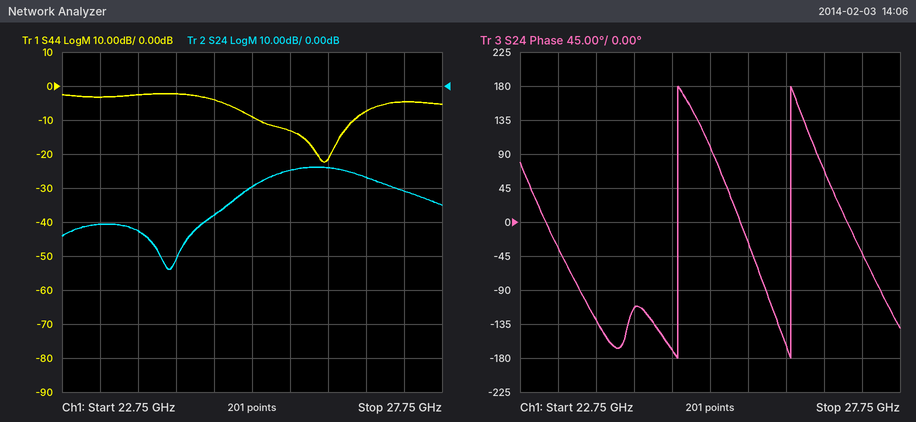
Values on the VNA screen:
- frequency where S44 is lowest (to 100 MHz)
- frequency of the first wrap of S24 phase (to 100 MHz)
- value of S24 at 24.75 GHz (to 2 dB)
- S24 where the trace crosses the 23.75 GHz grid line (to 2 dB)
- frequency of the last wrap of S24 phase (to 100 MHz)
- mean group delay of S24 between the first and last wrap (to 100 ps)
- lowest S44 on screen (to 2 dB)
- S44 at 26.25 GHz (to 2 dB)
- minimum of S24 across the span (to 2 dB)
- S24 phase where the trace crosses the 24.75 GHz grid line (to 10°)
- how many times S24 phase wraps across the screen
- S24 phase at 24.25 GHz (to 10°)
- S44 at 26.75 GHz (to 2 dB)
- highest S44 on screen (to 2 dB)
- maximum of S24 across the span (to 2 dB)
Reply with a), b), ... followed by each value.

a) 26.2 GHz
b) 24.8 GHz
c) -38 dB
d) -42 dB
e) 26.3 GHz
f) 700 ps
g) -22 dB
h) -22 dB
i) -54 dB
j) -170°
k) 2
l) -110°
m) -8 dB
n) -2 dB
o) -24 dB
